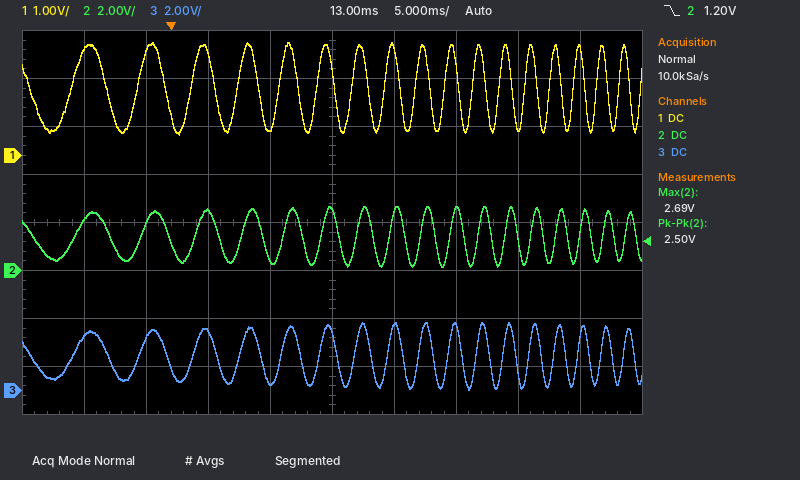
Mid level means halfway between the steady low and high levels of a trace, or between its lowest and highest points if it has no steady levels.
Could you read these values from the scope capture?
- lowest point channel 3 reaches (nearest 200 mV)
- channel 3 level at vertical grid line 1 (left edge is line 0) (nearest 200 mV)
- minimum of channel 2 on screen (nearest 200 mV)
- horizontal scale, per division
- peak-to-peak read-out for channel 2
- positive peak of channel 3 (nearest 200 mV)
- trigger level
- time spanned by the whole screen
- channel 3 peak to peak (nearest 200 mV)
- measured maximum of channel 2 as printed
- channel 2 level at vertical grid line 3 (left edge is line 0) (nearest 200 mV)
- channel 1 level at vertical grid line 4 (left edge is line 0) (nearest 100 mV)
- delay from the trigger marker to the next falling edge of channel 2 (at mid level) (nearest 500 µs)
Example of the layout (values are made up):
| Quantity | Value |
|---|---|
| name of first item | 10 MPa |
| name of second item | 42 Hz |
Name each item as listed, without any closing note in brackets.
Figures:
| Quantity | Value |
|---|---|
| lowest point channel 3 reaches | 0.0 V |
| channel 3 level at vertical grid line 1 (left edge is line 0) | 2.2 V |
| minimum of channel 2 on screen | 200 mV |
| horizontal scale, per division | 5 ms |
| peak-to-peak read-out for channel 2 | 2.50 V |
| positive peak of channel 3 | 2.8 V |
| trigger level | 1.20 V |
| time spanned by the whole screen | 50 ms |
| channel 3 peak to peak | 2.8 V |
| measured maximum of channel 2 as printed | 2.69 V |
| channel 2 level at vertical grid line 3 (left edge is line 0) | 2.4 V |
| channel 1 level at vertical grid line 4 (left edge is line 0) | 600 mV |
| delay from the trigger marker to the next falling edge of channel 2 (at mid level) | 4.0 ms |
